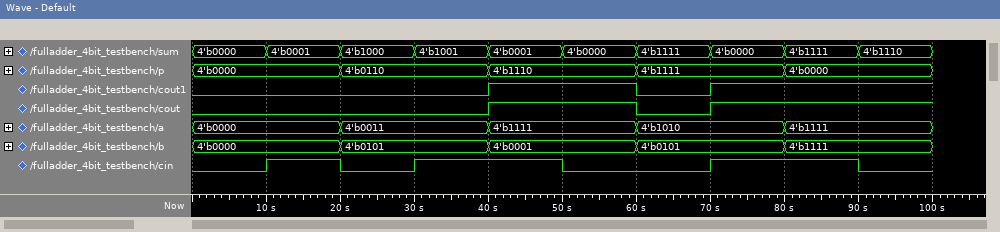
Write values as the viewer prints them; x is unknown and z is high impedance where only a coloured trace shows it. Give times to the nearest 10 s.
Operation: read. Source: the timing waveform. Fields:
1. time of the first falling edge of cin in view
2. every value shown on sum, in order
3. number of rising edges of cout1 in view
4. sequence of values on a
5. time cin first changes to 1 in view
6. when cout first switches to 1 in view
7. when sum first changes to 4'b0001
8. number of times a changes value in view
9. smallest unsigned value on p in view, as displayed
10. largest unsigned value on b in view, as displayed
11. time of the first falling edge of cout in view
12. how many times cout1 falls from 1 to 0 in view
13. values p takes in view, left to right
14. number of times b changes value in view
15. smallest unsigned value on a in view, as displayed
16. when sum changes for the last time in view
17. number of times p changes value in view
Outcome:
20 s
4'b0000, 4'b0001, 4'b1000, 4'b1001, 4'b0001, 4'b0000, 4'b1111, 4'b0000, 4'b1111, 4'b1110
2
4'b0000, 4'b0011, 4'b1111, 4'b1010, 4'b1111
10 s
40 s
10 s
4
4'b0000
4'b1111
60 s
1
4'b0000, 4'b0110, 4'b1110, 4'b1111, 4'b0000
4
4'b0000
90 s
4
